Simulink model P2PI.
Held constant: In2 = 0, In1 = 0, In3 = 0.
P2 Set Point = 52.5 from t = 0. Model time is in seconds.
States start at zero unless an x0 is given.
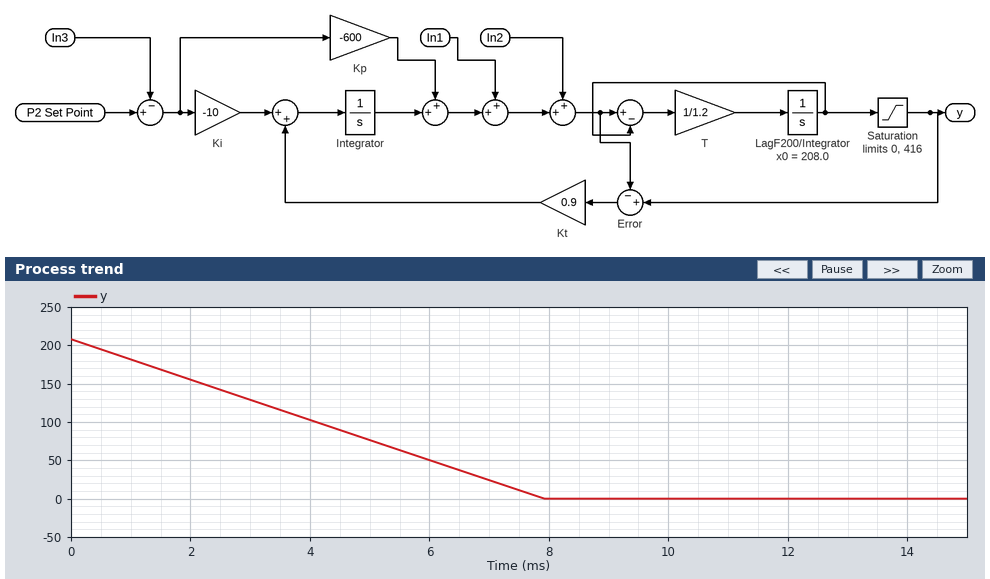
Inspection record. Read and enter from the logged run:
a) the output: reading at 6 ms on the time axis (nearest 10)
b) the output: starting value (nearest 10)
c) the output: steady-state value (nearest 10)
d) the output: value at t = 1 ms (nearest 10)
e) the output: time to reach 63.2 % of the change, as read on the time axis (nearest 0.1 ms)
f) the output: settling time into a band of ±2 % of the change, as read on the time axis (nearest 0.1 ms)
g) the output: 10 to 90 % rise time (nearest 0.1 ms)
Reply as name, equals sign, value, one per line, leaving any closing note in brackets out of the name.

the output: reading at 6 ms on the time axis = 50
the output: starting value = 210
the output: steady-state value = 0
the output: value at t = 1 ms = 180
the output: time to reach 63.2 % of the change, as read on the time axis = 5.0 ms
the output: settling time into a band of ±2 % of the change, as read on the time axis = 7.8 ms
the output: 10 to 90 % rise time = 6.3 ms
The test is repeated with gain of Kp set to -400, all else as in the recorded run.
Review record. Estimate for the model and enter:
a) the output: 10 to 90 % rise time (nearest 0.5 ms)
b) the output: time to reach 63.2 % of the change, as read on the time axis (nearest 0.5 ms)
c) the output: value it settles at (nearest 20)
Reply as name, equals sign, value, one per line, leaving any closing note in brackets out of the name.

the output: 10 to 90 % rise time = 9.5 ms
the output: time to reach 63.2 % of the change, as read on the time axis = 7.5 ms
the output: value it settles at = 0
